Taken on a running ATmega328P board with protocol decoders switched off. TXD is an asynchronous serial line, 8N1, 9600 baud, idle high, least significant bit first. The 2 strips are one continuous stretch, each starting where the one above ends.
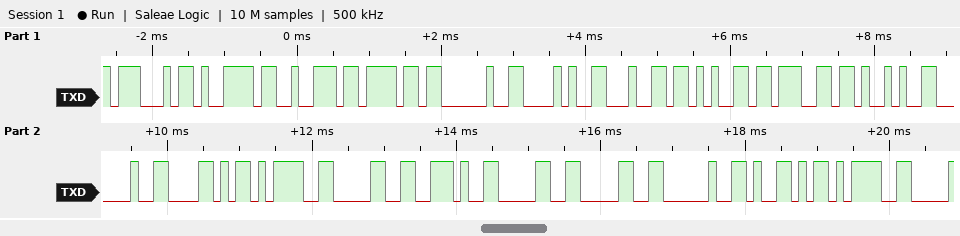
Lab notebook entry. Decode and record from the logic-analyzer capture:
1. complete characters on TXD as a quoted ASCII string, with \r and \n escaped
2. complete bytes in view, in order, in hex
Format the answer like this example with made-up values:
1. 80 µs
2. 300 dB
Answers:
1. "Gyro (deg) X=0.00 Y="
2. 47 79 72 6F 20 28 64 65 67 29 20 58 3D 30 2E 30 30 20 59 3D
